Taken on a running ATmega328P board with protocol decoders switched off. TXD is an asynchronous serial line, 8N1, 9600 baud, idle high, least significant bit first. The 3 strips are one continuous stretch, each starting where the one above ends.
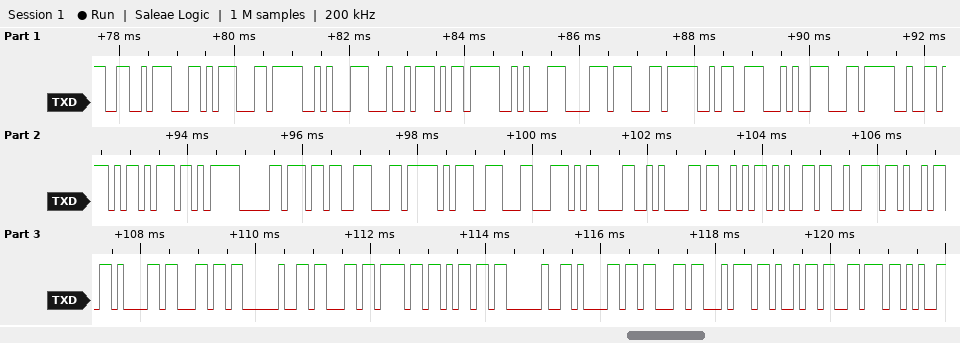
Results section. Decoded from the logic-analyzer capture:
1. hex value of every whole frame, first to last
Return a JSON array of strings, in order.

["A6 AC EC 8A A4 ED 8A B8 EC 9A 94 EC B2 AD EB B0 9B EC 9D 8C 0D 0A 53 65 72 69 61 6C 20 63 6F 6D 20 61 63 74 69 76"]
